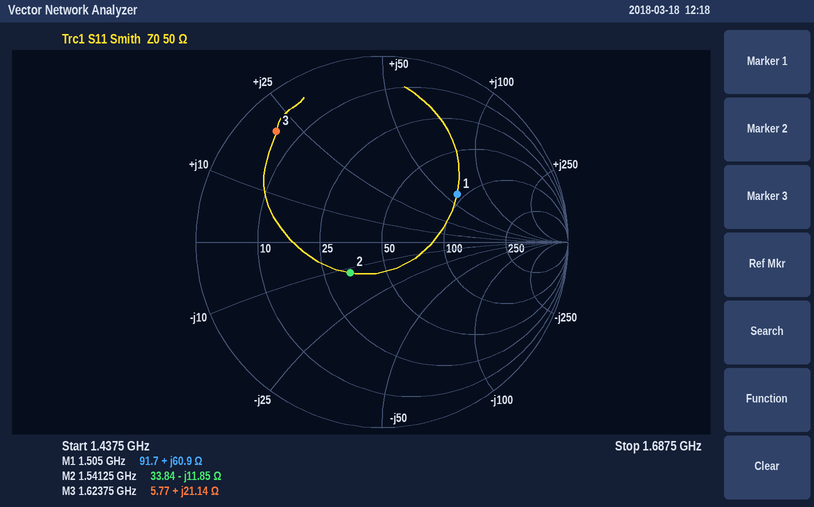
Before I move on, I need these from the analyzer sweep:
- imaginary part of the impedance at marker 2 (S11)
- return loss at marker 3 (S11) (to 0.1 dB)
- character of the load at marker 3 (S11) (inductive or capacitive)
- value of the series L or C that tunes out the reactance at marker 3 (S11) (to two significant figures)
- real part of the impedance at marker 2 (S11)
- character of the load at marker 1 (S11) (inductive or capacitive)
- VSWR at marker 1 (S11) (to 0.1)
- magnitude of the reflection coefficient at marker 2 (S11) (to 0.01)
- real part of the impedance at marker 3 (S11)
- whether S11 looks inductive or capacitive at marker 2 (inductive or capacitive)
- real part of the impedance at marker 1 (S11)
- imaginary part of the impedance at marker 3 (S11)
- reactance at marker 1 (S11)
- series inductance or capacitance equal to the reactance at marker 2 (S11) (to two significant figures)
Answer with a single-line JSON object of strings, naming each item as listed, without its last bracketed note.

{"imaginary part of the impedance at marker 2": "-11.85 Ω", "return loss at marker 3 (S11)": "1.7 dB", "character of the load at marker 3 (S11)": "inductive", "value of the series L or C that tunes out the reactance at marker 3 (S11)": "4.6 pF", "real part of the impedance at marker 2": "33.84 Ω", "character of the load at marker 1 (S11)": "inductive", "VSWR at marker 1 (S11)": "2.8", "magnitude of the reflection coefficient at marker 2 (S11)": "0.24", "real part of the impedance at marker 3": "5.77 Ω", "whether S11 looks inductive or capacitive at marker 2": "capacitive", "real part of the impedance at marker 1": "91.7 Ω", "imaginary part of the impedance at marker 3": "+21.14 Ω", "reactance at marker 1": "+60.9 Ω", "series inductance or capacitance equal to the reactance at marker 2 (S11)": "8.7 pF"}
